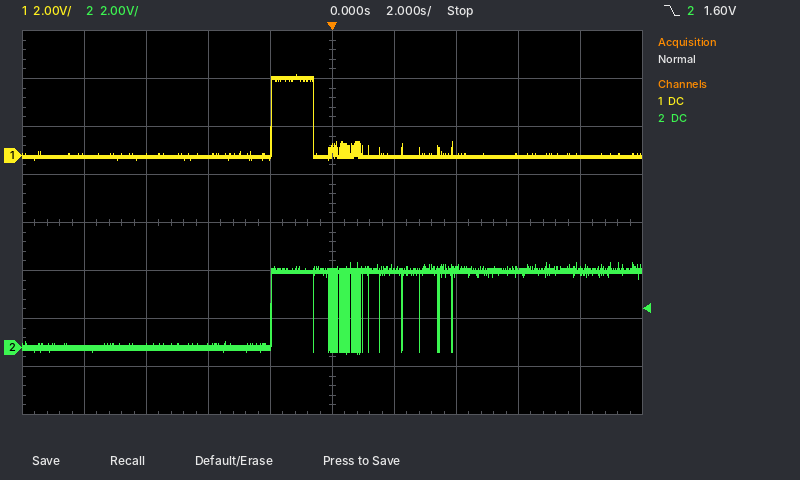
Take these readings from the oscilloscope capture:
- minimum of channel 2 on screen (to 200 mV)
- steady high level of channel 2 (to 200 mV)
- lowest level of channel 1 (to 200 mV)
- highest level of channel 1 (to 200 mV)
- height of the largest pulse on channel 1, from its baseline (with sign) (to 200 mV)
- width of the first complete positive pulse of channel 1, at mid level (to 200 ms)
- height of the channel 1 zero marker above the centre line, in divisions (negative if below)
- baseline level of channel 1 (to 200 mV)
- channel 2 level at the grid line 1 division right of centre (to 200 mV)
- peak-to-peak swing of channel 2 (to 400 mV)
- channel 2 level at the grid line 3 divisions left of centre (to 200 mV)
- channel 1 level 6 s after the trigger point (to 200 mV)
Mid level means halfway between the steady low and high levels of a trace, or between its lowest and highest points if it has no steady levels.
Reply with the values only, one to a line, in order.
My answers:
-200 mV
3.2 V
-200 mV
3.4 V
+3.4 V
1.4 s
+1.4 div
0.0 V
3.2 V
3.6 V
0.0 V
0.0 V
